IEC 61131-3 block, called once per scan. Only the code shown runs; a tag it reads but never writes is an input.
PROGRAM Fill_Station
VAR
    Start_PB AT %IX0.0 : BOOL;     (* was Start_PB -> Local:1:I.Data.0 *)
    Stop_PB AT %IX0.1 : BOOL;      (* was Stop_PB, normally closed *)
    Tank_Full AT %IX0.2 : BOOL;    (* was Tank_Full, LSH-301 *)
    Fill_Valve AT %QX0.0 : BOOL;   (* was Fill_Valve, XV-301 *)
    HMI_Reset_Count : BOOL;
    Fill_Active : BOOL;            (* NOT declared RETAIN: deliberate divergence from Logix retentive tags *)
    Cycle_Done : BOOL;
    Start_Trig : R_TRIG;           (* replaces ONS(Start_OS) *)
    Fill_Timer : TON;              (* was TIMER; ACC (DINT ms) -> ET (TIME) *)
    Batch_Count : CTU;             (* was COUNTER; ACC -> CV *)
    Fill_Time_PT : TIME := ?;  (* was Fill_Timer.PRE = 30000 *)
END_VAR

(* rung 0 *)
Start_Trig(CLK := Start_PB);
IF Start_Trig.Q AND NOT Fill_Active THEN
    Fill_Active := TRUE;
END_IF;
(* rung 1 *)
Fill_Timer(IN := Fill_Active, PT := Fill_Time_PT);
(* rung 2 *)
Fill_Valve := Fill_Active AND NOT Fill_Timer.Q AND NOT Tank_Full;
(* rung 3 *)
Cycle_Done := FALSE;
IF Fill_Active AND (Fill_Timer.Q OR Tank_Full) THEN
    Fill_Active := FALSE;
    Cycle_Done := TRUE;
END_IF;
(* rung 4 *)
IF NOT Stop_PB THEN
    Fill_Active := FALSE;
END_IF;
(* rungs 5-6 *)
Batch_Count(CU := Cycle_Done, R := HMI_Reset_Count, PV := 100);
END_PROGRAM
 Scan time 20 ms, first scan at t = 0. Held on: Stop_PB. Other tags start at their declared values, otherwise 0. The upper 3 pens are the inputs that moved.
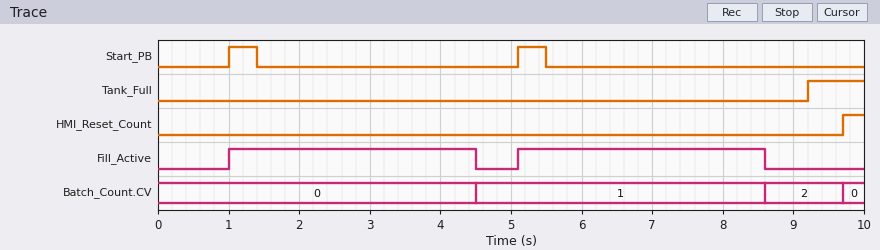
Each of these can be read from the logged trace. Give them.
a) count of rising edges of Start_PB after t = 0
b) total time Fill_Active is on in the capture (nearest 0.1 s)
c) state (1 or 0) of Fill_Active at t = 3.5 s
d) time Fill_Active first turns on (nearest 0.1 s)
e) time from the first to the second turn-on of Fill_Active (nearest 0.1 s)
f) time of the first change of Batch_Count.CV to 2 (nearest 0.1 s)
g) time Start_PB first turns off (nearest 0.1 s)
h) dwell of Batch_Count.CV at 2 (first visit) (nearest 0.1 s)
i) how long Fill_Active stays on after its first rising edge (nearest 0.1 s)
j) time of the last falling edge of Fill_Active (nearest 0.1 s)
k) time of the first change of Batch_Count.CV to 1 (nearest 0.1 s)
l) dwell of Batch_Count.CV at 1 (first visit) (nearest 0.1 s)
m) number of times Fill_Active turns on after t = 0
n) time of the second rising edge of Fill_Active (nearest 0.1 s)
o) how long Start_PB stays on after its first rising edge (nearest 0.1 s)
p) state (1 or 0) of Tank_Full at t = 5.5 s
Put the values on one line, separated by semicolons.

2; 7.0 s; 1; 1.0 s; 4.1 s; 8.6 s; 1.4 s; 1.1 s; 3.5 s; 8.6 s; 4.5 s; 4.1 s; 2; 5.1 s; 0.4 s; 0
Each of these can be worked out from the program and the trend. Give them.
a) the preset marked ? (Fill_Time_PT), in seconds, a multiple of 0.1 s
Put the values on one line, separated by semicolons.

3.5 s
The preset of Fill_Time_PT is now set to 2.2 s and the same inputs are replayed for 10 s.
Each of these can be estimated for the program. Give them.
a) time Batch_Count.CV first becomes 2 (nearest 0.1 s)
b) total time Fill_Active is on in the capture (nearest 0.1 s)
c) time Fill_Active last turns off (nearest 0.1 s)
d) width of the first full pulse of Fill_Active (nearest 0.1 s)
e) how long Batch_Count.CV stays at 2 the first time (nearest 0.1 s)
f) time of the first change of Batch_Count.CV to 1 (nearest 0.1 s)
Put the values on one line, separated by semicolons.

7.3 s; 4.4 s; 7.3 s; 2.2 s; 2.4 s; 3.2 s
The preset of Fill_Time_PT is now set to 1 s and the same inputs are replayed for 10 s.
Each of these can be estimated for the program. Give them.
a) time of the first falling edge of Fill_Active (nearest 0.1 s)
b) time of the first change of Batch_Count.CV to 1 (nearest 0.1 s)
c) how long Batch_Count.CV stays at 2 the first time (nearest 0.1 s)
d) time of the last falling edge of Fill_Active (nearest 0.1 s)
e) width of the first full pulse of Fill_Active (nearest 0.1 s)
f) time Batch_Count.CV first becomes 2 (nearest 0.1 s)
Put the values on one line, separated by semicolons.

2.0 s; 2.0 s; 3.6 s; 6.1 s; 1.0 s; 6.1 s
